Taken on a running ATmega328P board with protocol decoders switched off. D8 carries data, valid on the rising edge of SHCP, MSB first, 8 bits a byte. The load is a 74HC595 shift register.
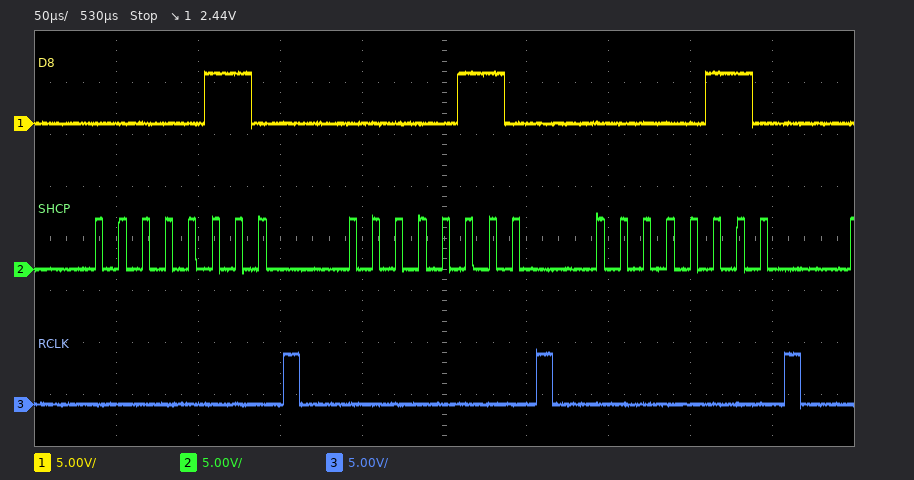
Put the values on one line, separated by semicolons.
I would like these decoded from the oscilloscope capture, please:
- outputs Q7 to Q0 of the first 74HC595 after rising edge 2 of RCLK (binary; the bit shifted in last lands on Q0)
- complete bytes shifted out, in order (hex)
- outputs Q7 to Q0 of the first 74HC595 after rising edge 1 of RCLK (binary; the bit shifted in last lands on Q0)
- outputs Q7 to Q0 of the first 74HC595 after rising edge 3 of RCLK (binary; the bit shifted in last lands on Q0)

00000110; 0x06 0x06 0x06; 00000110; 00000110
